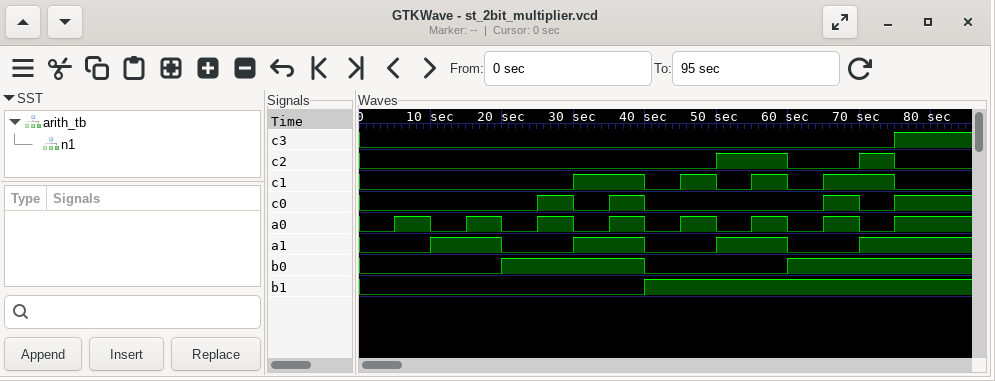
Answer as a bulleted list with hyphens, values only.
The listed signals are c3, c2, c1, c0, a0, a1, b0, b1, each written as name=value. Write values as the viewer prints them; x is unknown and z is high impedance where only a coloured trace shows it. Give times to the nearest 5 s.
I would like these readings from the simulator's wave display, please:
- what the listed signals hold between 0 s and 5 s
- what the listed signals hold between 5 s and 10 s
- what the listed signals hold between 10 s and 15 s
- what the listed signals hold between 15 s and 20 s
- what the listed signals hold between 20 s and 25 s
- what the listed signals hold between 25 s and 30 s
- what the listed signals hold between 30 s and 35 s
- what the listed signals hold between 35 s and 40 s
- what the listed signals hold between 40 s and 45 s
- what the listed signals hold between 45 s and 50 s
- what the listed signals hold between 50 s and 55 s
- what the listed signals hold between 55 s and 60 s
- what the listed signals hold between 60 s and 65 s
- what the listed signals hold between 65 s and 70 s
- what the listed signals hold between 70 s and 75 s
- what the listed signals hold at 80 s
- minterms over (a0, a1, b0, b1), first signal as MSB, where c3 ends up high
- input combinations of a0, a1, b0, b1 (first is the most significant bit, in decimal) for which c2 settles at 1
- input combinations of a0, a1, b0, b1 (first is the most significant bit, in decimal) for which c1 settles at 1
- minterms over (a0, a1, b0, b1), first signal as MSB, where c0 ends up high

- c3=0, c2=0, c1=0, c0=0, a0=0, a1=0, b0=0, b1=0
- c3=0, c2=0, c1=0, c0=0, a0=1, a1=0, b0=0, b1=0
- c3=0, c2=0, c1=0, c0=0, a0=0, a1=1, b0=0, b1=0
- c3=0, c2=0, c1=0, c0=0, a0=1, a1=1, b0=0, b1=0
- c3=0, c2=0, c1=0, c0=0, a0=0, a1=0, b0=1, b1=0
- c3=0, c2=0, c1=0, c0=1, a0=1, a1=0, b0=1, b1=0
- c3=0, c2=0, c1=1, c0=0, a0=0, a1=1, b0=1, b1=0
- c3=0, c2=0, c1=1, c0=1, a0=1, a1=1, b0=1, b1=0
- c3=0, c2=0, c1=0, c0=0, a0=0, a1=0, b0=0, b1=1
- c3=0, c2=0, c1=1, c0=0, a0=1, a1=0, b0=0, b1=1
- c3=0, c2=1, c1=0, c0=0, a0=0, a1=1, b0=0, b1=1
- c3=0, c2=1, c1=1, c0=0, a0=1, a1=1, b0=0, b1=1
- c3=0, c2=0, c1=0, c0=0, a0=0, a1=0, b0=1, b1=1
- c3=0, c2=0, c1=1, c0=1, a0=1, a1=0, b0=1, b1=1
- c3=0, c2=1, c1=1, c0=0, a0=0, a1=1, b0=1, b1=1
- c3=1, c2=0, c1=0, c0=1, a0=1, a1=1, b0=1, b1=1
- 15
- 5, 7, 13
- 6, 7, 9, 11, 13, 14
- 10, 11, 14, 15
